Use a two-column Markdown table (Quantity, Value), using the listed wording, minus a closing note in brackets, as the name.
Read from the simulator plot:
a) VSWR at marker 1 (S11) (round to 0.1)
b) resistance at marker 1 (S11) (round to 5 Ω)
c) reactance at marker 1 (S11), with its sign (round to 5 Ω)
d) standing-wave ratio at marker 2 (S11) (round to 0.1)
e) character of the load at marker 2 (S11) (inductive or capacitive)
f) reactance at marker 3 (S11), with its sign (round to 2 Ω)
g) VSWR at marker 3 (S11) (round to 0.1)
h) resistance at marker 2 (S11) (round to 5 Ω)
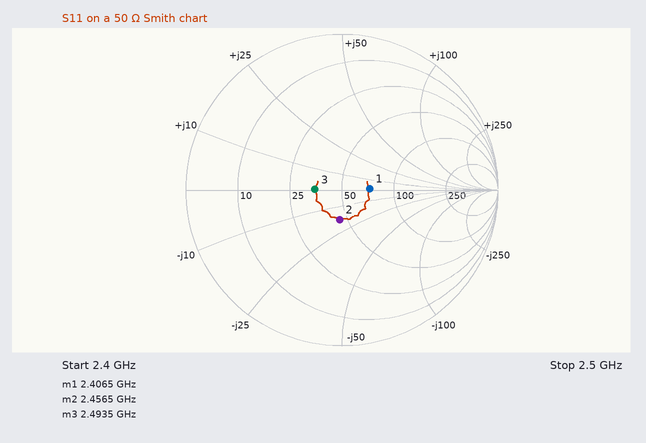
| Quantity | Value |
|---|---|
| VSWR at marker 1 (S11) | 1.4 |
| resistance at marker 1 (S11) | 70 Ω |
| reactance at marker 1 (S11), with its sign | 0 Ω |
| standing-wave ratio at marker 2 (S11) | 1.5 |
| character of the load at marker 2 (S11) | capacitive |
| reactance at marker 3 (S11), with its sign | 0 Ω |
| VSWR at marker 3 (S11) | 1.4 |
| resistance at marker 2 (S11) | 45 Ω |
